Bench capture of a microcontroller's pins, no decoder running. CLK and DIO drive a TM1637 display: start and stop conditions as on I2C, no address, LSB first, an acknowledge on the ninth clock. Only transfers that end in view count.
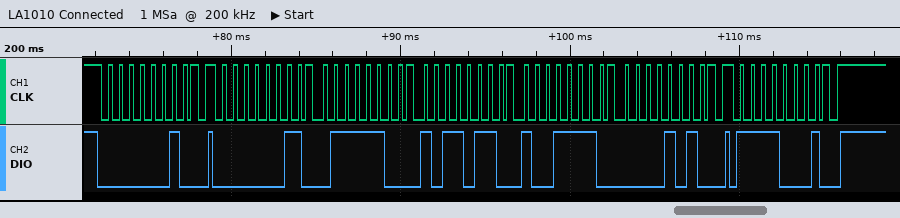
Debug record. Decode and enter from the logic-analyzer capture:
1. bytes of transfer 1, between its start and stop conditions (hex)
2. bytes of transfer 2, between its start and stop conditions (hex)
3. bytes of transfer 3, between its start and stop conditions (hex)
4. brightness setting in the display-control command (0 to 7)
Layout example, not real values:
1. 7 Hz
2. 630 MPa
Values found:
1. 40
2. C0 3E 6D 79 50
3. 8F
4. 7
